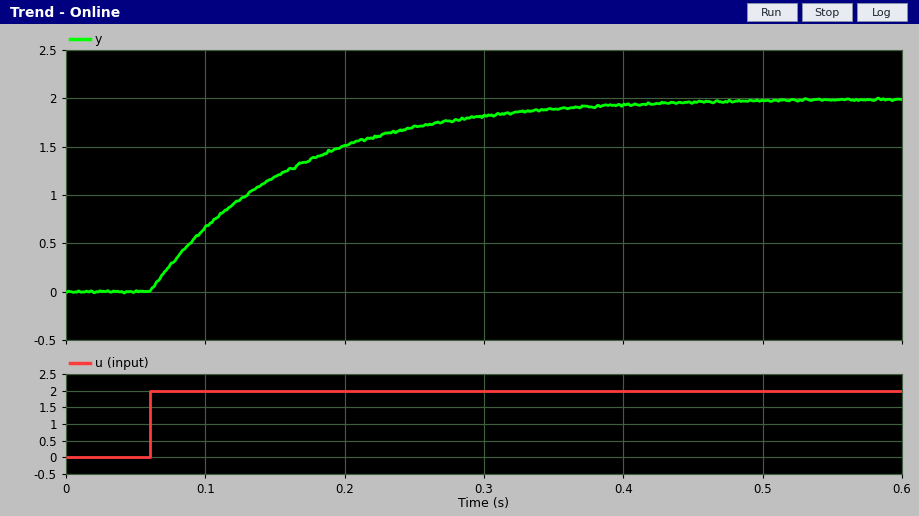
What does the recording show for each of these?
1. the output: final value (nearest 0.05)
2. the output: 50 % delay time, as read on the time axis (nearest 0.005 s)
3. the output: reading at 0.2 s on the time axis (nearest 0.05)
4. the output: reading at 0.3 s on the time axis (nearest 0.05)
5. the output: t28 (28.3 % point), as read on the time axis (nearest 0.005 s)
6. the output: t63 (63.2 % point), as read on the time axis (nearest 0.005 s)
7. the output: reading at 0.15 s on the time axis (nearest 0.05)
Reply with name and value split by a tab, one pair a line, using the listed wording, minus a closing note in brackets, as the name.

the output: final value	2.00
the output: 50 % delay time, as read on the time axis	0.130 s
the output: reading at 0.2 s on the time axis	1.50
the output: reading at 0.3 s on the time axis	1.80
the output: t28 (28.3 % point), as read on the time axis	0.095 s
the output: t63 (63.2 % point), as read on the time axis	0.160 s
the output: reading at 0.15 s on the time axis	1.20
